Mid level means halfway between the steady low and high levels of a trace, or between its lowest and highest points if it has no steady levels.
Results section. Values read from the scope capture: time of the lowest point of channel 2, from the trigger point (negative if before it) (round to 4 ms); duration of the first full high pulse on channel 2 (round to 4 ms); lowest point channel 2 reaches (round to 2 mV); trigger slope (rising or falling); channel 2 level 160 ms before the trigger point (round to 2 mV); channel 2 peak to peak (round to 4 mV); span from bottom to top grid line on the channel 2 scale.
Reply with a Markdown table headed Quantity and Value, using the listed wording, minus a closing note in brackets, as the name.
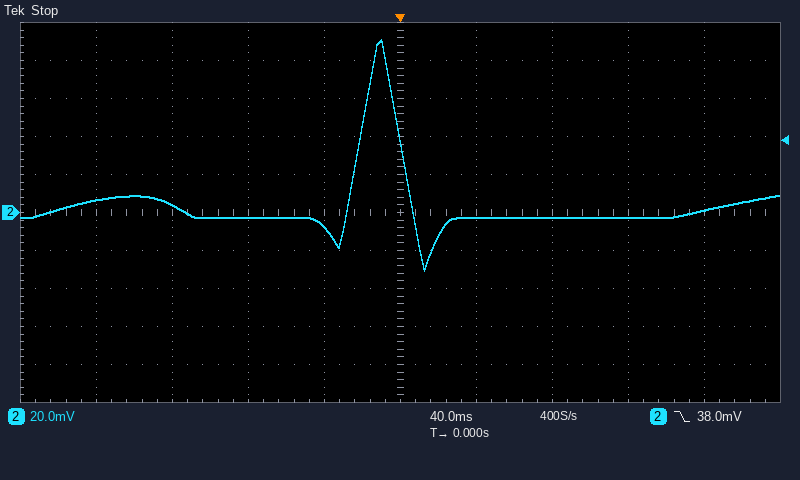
| Quantity | Value |
|---|---|
| time of the lowest point of channel 2, from the trigger point (negative if before it) | +12 ms |
| duration of the first full high pulse on channel 2 | 24 ms |
| lowest point channel 2 reaches | -30 mV |
| trigger slope | falling |
| channel 2 level 160 ms before the trigger point | 6 mV |
| channel 2 peak to peak | 120 mV |
| span from bottom to top grid line on the channel 2 scale | 200 mV |
